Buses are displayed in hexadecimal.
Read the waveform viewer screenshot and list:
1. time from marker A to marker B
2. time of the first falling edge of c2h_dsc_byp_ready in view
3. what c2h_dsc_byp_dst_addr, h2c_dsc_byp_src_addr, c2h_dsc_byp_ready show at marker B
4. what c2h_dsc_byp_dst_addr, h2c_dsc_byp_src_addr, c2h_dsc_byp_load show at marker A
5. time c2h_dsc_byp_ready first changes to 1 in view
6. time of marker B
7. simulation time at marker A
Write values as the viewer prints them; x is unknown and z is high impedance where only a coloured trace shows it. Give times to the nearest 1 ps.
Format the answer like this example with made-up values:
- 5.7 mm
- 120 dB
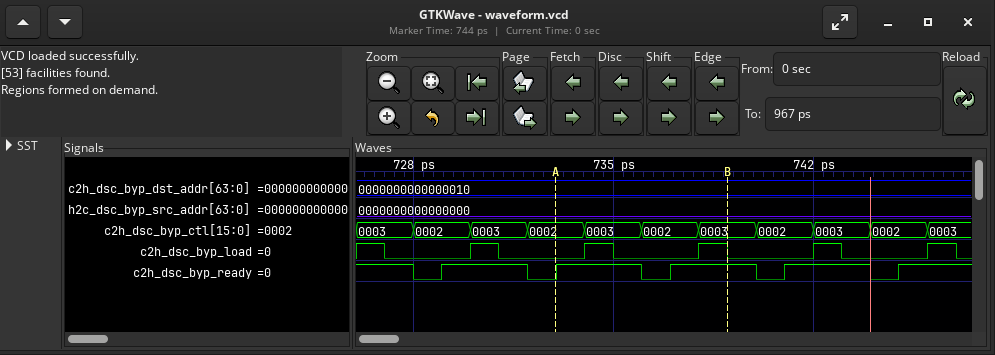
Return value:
- 6 ps
- 728 ps
- c2h_dsc_byp_dst_addr=0000000000000010, h2c_dsc_byp_src_addr=0000000000000000, c2h_dsc_byp_ready=1
- c2h_dsc_byp_dst_addr=0000000000000010, h2c_dsc_byp_src_addr=0000000000000000, c2h_dsc_byp_load=0
- 729 ps
- 739 ps
- 733 ps
